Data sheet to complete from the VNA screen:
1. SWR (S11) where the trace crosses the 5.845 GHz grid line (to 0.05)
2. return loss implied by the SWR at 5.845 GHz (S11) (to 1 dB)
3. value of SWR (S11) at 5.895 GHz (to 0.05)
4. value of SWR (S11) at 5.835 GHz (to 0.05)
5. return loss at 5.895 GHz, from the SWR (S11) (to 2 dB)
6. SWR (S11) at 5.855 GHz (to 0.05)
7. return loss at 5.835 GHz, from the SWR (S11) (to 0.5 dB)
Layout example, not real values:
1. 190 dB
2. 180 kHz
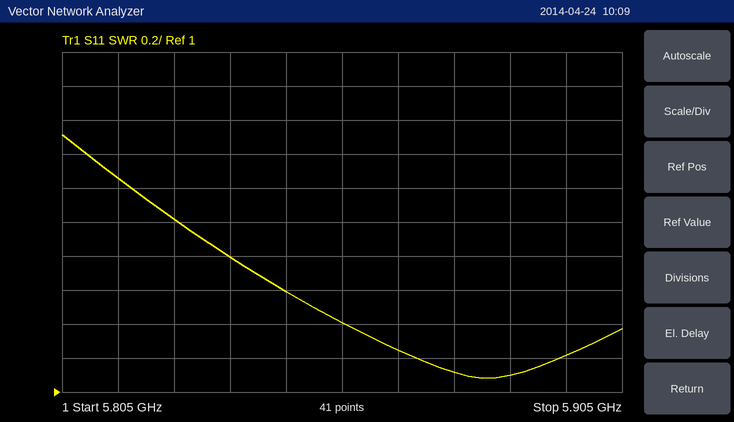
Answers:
1. 1.60
2. 13 dB
3. 1.20
4. 1.80
5. 20 dB
6. 1.40
7. 11.0 dB
